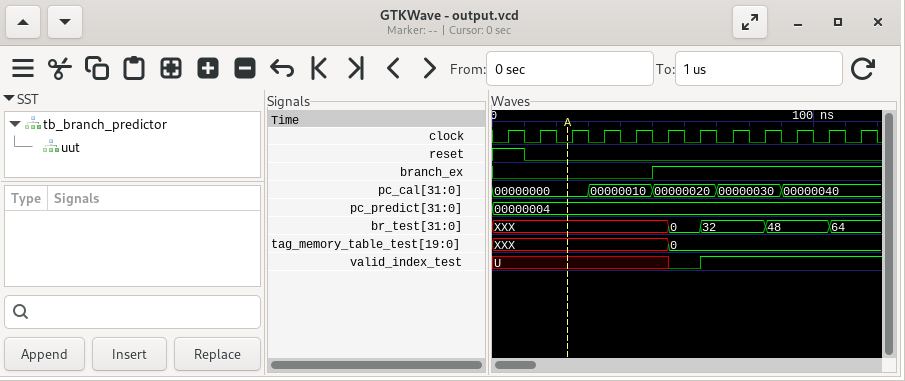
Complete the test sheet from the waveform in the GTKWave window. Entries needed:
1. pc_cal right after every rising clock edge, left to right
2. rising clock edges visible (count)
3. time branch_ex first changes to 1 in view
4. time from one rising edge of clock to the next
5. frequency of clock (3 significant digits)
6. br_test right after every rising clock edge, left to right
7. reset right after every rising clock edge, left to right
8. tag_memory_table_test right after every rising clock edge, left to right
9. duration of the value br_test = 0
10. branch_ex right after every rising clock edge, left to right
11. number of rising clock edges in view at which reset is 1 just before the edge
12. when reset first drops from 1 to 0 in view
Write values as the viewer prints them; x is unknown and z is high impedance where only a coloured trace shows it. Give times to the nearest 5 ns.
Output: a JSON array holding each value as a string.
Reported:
["00000000, 00000000, 00000000, 00000010, 00000010, 00000020, 00000020, 00000030, 00000030, 00000040, 00000040, 00000040", "12", "50 ns", "10 ns", "100 MHz", "XXX, XXX, XXX, XXX, XXX, 0, 32, 32, 48, 48, 64, 64", "1 0 0 0 0 0 0 0 0 0 0 0", "XXX, XXX, XXX, XXX, XXX, 0, 0, 0, 0, 0, 0, 0", "10 ns", "0 0 0 0 0 1 1 1 1 1 1 1", "1", "10 ns"]
